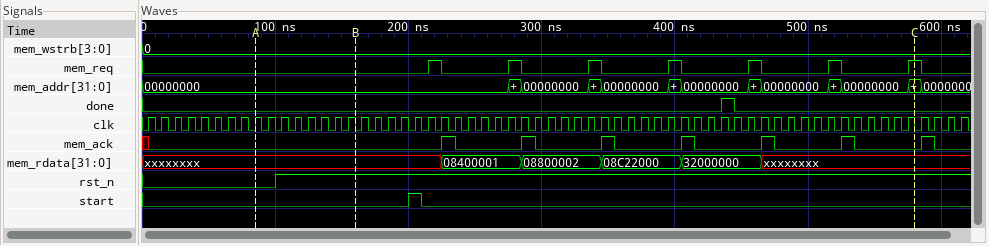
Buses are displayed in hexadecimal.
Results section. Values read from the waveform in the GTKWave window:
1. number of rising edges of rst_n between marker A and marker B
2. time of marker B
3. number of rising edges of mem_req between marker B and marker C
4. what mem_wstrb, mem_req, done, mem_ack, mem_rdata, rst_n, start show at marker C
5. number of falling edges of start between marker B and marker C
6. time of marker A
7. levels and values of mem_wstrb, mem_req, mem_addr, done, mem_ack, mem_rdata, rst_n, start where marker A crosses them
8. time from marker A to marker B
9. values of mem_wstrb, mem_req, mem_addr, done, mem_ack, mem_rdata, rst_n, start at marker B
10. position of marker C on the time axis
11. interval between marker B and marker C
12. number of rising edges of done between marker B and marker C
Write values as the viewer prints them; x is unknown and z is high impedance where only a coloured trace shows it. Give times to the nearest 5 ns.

1
160 ns
7
mem_wstrb=0, mem_req=1, done=0, mem_ack=0, mem_rdata=xxxxxxxx, rst_n=1, start=0
1
85 ns
mem_wstrb=0, mem_req=0, mem_addr=00000000, done=0, mem_ack=0, mem_rdata=xxxxxxxx, rst_n=0, start=0
75 ns
mem_wstrb=0, mem_req=0, mem_addr=00000000, done=0, mem_ack=0, mem_rdata=xxxxxxxx, rst_n=1, start=0
580 ns
420 ns
1
